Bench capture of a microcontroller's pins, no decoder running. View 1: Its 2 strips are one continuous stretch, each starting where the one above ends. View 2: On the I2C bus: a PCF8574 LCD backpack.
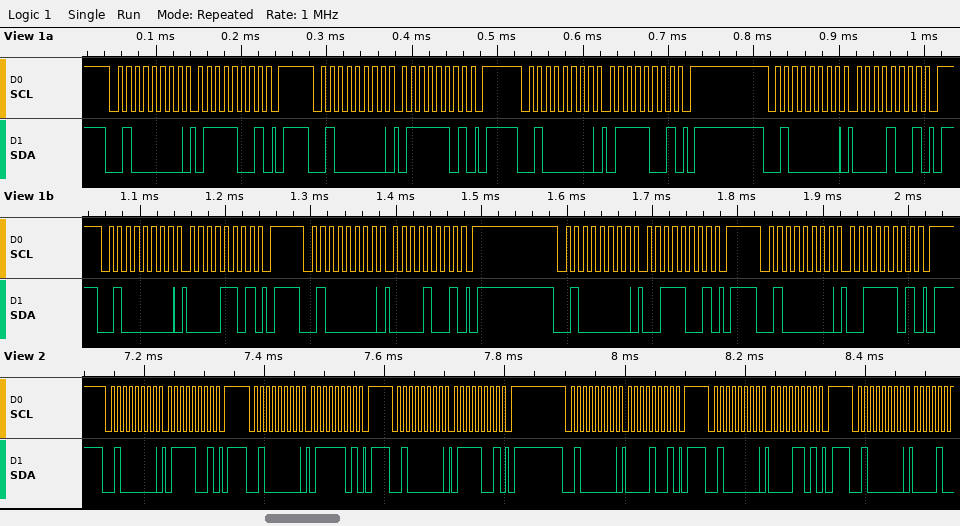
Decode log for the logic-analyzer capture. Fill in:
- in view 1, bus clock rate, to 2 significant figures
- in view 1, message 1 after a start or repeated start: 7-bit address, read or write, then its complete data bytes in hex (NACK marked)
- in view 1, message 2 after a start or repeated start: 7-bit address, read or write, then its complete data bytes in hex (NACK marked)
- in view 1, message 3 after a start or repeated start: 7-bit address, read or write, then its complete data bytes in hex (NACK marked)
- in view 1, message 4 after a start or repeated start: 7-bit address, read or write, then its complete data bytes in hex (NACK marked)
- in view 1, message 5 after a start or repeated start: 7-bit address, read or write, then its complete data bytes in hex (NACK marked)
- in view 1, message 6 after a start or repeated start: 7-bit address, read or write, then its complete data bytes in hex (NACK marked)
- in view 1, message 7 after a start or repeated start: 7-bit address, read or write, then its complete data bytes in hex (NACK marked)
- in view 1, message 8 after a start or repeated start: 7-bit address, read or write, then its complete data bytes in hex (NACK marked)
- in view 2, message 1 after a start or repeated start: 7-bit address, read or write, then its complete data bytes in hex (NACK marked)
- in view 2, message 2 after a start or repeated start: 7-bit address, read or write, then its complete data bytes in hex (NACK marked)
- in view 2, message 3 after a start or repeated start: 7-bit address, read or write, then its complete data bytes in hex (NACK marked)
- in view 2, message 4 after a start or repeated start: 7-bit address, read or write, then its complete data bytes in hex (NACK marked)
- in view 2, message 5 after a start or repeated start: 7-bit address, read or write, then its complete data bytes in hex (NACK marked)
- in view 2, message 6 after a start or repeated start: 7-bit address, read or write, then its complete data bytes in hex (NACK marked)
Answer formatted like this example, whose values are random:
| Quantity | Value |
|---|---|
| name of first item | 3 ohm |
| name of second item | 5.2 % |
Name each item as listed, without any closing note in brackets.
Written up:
| Quantity | Value |
|---|---|
| in view 1, bus clock rate, to 2 significant figures | 100 kHz |
| in view 1, message 1 after a start or repeated start: 7-bit address, read or write, then its complete data bytes in hex | 0x20 write: 79 |
| in view 1, message 2 after a start or repeated start: 7-bit address, read or write, then its complete data bytes in hex | 0x20 write: 7D |
| in view 1, message 3 after a start or repeated start: 7-bit address, read or write, then its complete data bytes in hex | 0x20 write: 79 |
| in view 1, message 4 after a start or repeated start: 7-bit address, read or write, then its complete data bytes in hex | 0x20 write: 09 |
| in view 1, message 5 after a start or repeated start: 7-bit address, read or write, then its complete data bytes in hex | 0x20 write: 0D |
| in view 1, message 6 after a start or repeated start: 7-bit address, read or write, then its complete data bytes in hex | 0x20 write: 09 |
| in view 1, message 7 after a start or repeated start: 7-bit address, read or write, then its complete data bytes in hex | 0x20 write: 39 |
| in view 1, message 8 after a start or repeated start: 7-bit address, read or write, then its complete data bytes in hex | 0x20 write: 3D |
| in view 2, message 1 after a start or repeated start: 7-bit address, read or write, then its complete data bytes in hex | 0x20 write: 79 |
| in view 2, message 2 after a start or repeated start: 7-bit address, read or write, then its complete data bytes in hex | 0x20 write: 7D |
| in view 2, message 3 after a start or repeated start: 7-bit address, read or write, then its complete data bytes in hex | 0x20 write: 79 |
| in view 2, message 4 after a start or repeated start: 7-bit address, read or write, then its complete data bytes in hex | 0x20 write: 09 |
| in view 2, message 5 after a start or repeated start: 7-bit address, read or write, then its complete data bytes in hex | 0x20 write: 0D |
| in view 2, message 6 after a start or repeated start: 7-bit address, read or write, then its complete data bytes in hex | 0x20 write |
